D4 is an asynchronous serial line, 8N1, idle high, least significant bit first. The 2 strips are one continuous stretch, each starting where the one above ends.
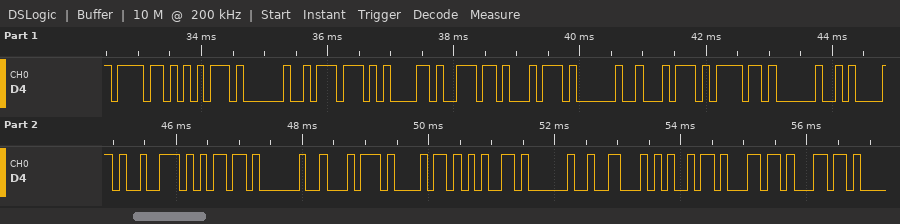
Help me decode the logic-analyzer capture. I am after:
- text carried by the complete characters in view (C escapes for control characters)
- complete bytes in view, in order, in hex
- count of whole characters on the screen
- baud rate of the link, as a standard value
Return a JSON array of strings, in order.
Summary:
["\"ou want to arm the Fill\"", "6F 75 20 77 61 6E 74 20 74 6F 20 61 72 6D 20 74 68 65 20 46 69 6C 6C", "23", "9600 baud"]
